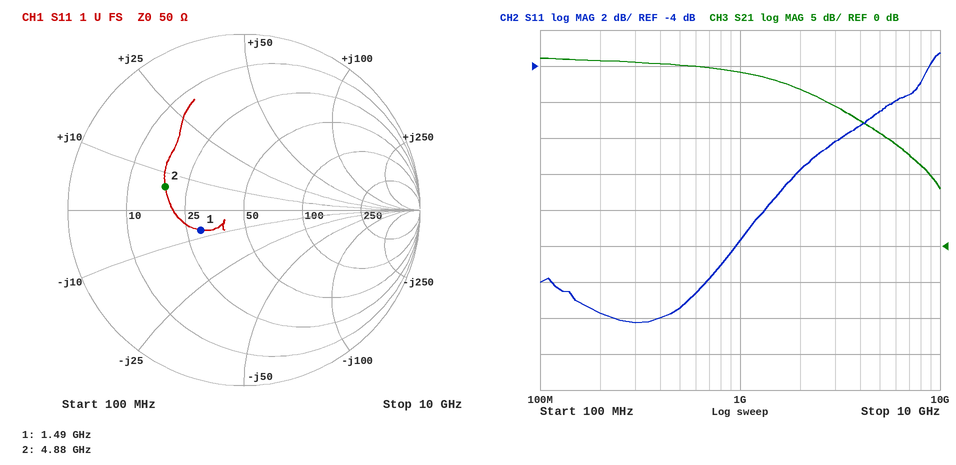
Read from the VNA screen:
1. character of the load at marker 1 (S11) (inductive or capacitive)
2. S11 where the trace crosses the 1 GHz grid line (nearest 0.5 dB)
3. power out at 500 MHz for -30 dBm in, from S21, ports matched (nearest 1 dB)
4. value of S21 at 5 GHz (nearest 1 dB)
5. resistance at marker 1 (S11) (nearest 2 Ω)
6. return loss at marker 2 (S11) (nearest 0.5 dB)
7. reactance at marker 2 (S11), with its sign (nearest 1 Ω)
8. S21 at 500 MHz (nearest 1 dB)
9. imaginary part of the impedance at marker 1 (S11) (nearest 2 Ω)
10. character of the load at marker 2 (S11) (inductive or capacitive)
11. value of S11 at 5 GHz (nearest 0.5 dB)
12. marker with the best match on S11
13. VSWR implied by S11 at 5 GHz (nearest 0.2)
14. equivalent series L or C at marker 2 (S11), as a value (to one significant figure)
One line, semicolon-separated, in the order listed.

capacitive; -13.5 dB; -5 dBm; 16 dB; 30 Ω; 6.5 dB; +6 Ω; 25 dB; -8 Ω; inductive; -6.5 dB; marker 1; 2.8; 200 pH
